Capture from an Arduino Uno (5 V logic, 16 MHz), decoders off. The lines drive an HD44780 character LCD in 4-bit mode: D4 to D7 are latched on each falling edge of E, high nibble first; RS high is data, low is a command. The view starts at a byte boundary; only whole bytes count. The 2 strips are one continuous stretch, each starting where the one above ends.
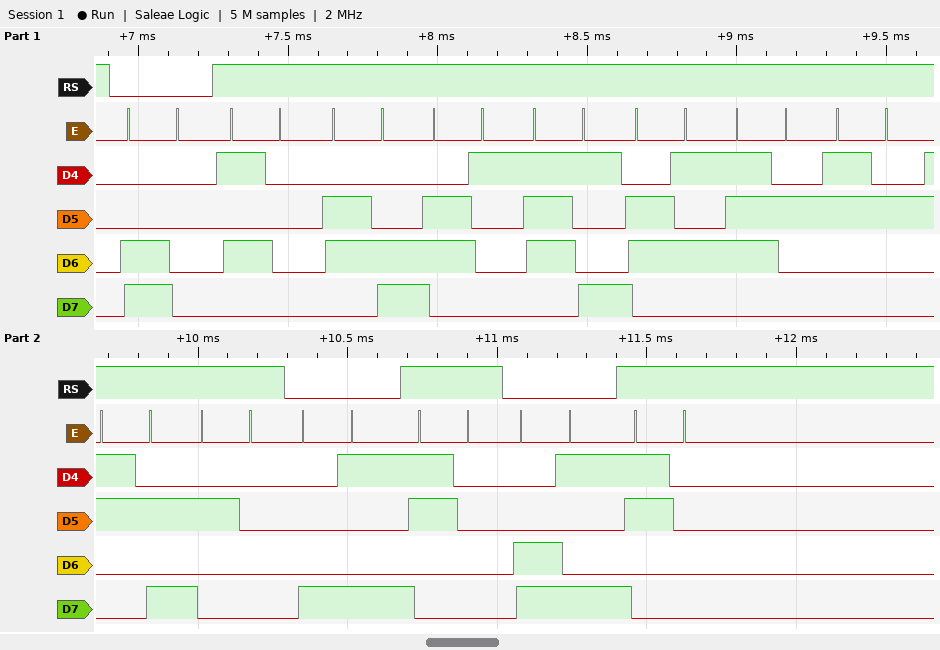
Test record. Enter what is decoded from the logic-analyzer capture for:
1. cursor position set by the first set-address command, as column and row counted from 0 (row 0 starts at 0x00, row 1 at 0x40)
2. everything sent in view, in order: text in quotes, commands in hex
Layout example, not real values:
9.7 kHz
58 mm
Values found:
column 0, row 1
0xC0 "Player2: " 0x89 "0" 0xC9 "0"
